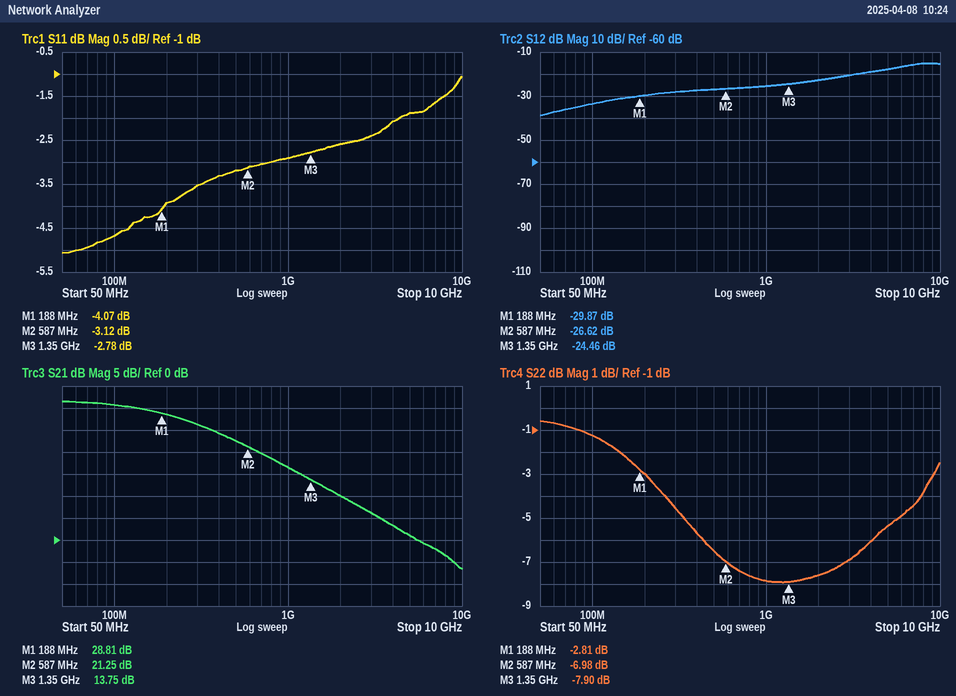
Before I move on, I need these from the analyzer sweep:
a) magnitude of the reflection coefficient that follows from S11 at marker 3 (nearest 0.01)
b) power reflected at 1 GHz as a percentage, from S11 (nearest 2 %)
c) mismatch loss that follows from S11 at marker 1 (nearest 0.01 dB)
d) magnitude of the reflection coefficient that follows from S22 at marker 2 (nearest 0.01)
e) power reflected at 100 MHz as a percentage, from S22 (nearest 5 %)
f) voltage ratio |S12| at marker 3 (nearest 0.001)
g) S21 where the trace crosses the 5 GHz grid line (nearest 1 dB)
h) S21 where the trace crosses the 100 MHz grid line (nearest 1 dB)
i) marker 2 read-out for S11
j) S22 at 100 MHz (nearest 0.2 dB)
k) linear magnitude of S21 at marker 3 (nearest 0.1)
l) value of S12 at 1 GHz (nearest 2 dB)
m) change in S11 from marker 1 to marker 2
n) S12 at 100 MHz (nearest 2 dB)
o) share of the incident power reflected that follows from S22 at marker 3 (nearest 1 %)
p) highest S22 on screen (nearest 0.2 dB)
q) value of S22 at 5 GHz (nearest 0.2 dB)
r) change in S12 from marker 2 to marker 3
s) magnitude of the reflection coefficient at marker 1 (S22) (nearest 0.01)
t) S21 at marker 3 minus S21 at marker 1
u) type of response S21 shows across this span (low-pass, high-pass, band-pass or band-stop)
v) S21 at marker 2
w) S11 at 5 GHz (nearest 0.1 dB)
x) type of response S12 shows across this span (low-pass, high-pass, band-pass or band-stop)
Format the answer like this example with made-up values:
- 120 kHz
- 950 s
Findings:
- 0.73
- 52 %
- 2.16 dB
- 0.45
- 75 %
- 0.060
- 1 dB
- 31 dB
- -3.12 dB
- -1.2 dB
- 4.9
- -26 dB
- 0.95 dB
- -34 dB
- 16 %
- -0.6 dB
- -5.4 dB
- 2.16 dB
- 0.72
- -15.06 dB
- low-pass
- 21.25 dB
- -1.9 dB
- high-pass
